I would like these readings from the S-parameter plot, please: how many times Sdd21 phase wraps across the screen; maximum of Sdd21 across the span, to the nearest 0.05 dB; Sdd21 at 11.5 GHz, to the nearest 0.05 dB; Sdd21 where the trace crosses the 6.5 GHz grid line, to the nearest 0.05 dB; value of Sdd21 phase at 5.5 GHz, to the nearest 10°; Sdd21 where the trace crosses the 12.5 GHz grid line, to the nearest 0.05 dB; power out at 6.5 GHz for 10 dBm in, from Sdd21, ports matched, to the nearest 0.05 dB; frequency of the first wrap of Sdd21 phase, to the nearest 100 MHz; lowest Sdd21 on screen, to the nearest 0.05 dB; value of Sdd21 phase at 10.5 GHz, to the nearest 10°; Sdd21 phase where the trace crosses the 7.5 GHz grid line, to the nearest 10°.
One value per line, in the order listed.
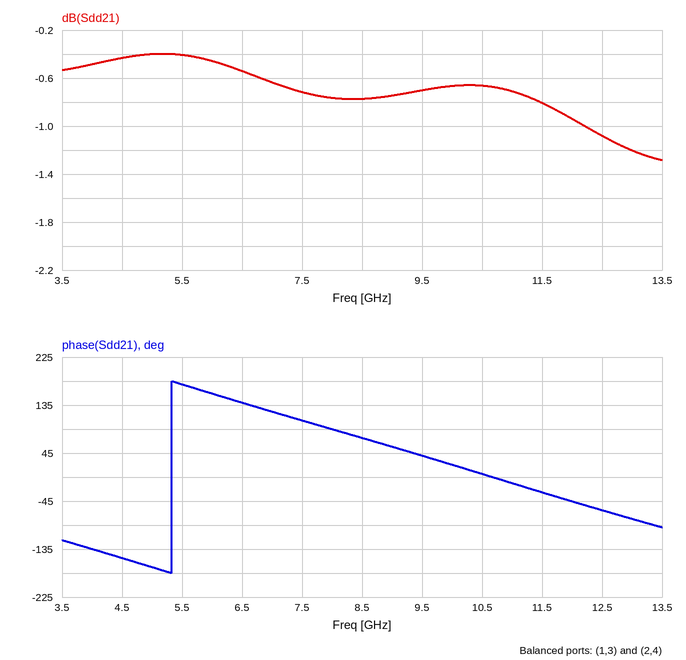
1
-0.40 dB
-0.80 dB
-0.55 dB
170°
-1.10 dB
9.45 dBm
5.3 GHz
-1.30 dB
10°
110°
